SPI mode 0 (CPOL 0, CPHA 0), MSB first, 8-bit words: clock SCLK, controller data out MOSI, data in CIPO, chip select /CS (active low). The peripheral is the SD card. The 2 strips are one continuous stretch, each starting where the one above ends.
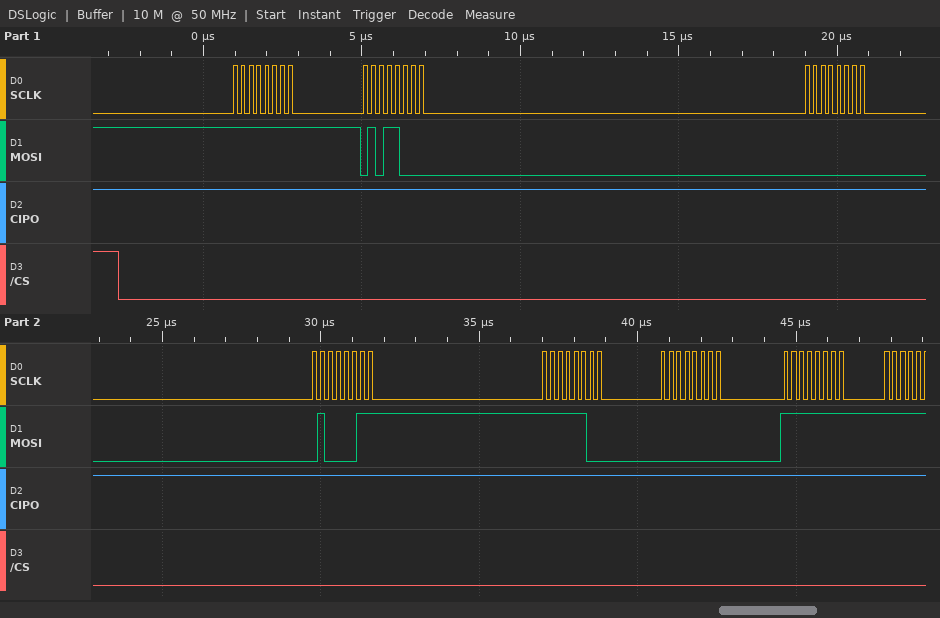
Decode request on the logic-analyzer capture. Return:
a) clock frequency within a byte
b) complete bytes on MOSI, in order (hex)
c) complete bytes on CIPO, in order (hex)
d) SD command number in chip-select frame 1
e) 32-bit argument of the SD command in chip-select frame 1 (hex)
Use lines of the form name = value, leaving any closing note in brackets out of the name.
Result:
clock frequency within a byte = 4 MHz
complete bytes on MOSI, in order = FF 58 00 43 FC 00 FF
complete bytes on CIPO, in order = FF FF FF FF FF FF FF
SD command number in chip-select frame 1 = CMD24
32-bit argument of the SD command in chip-select frame 1 = 0x0043FC00
